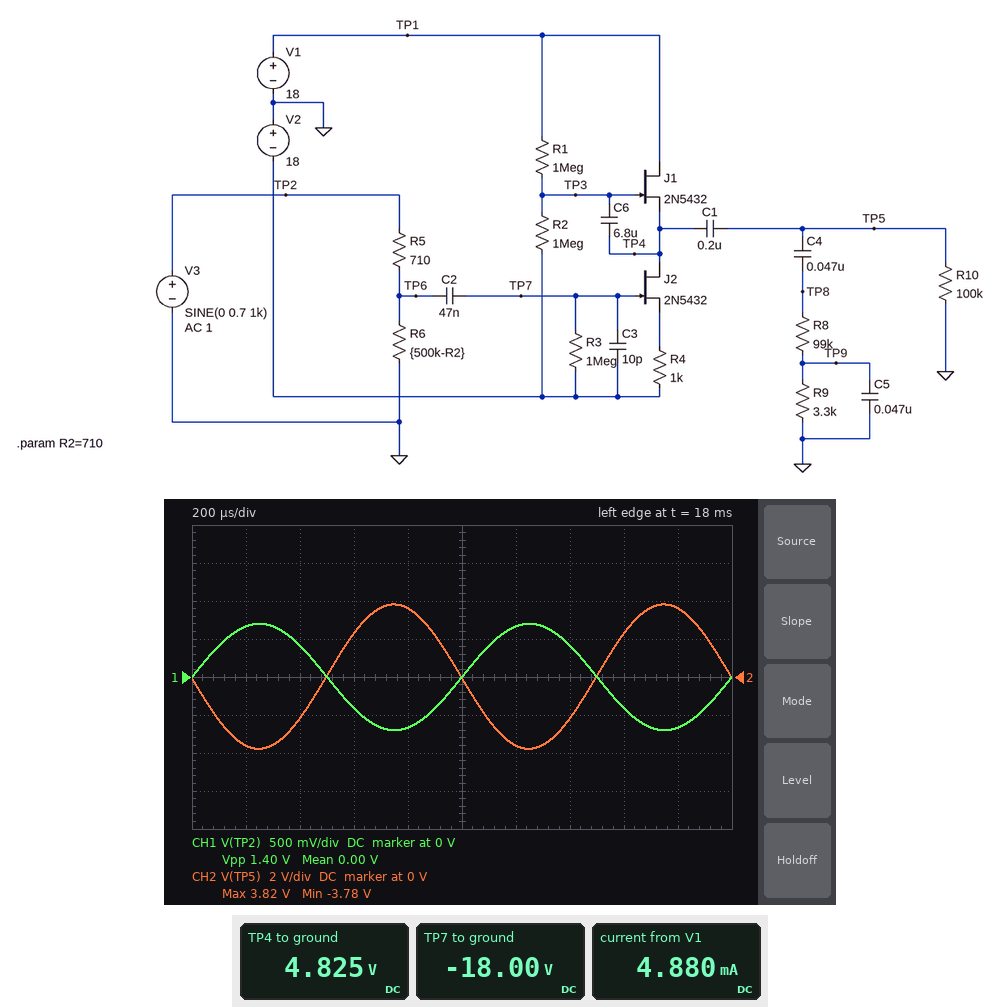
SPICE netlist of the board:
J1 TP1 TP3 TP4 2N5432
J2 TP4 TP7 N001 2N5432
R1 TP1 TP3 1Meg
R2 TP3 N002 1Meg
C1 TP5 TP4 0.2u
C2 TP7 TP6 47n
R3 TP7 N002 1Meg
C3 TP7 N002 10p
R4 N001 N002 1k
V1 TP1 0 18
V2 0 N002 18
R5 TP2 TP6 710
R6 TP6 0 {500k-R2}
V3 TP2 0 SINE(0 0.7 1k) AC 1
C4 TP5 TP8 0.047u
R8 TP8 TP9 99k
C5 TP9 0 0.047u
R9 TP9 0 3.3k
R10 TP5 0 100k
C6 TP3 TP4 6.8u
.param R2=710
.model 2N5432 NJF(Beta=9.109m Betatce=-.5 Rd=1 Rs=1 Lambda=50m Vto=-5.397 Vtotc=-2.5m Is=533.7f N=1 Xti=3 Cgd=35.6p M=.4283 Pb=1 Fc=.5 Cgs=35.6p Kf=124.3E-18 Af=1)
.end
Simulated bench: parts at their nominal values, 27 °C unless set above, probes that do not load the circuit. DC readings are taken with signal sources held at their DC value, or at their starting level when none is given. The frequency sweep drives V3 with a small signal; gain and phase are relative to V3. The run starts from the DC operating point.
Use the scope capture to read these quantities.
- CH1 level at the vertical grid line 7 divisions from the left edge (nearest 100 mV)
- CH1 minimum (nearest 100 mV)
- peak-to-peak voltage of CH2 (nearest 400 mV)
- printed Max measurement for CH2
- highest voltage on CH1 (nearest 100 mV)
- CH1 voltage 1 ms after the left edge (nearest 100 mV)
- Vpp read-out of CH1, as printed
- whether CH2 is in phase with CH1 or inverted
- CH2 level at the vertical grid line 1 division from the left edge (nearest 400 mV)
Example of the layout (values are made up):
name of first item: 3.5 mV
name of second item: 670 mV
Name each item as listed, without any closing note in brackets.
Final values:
CH1 level at the vertical grid line 7 divisions from the left edge: 400 mV
CH1 minimum: -700 mV
peak-to-peak voltage of CH2: 7.6 V
printed Max measurement for CH2: 3.82 V
highest voltage on CH1: 700 mV
CH1 voltage 1 ms after the left edge: 0 V
Vpp read-out of CH1, as printed: 1.40 V
whether CH2 is in phase with CH1 or inverted: inverted
CH2 level at the vertical grid line 1 division from the left edge: -3.6 V
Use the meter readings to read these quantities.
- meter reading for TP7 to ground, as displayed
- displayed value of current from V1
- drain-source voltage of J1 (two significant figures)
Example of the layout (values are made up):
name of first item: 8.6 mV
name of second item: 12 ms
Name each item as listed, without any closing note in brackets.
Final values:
meter reading for TP7 to ground, as displayed: -18.00 V
displayed value of current from V1: 4.880 mA
drain-source voltage of J1: 13 V
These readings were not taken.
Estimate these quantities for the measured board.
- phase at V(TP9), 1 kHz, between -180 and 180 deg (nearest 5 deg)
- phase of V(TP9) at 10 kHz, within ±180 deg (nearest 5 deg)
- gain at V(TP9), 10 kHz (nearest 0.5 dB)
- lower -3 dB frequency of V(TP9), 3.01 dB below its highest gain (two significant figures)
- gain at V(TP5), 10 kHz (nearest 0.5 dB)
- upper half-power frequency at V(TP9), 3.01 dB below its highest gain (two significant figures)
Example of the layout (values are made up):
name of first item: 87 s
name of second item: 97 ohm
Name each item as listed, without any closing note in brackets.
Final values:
phase at V(TP9), 1 kHz, between -180 and 180 deg: 140 deg
phase of V(TP9) at 10 kHz, within ±180 deg: 95 deg
gain at V(TP9), 10 kHz: -34.5 dB
lower -3 dB frequency of V(TP9), 3.01 dB below its highest gain: 38 Hz
gain at V(TP5), 10 kHz: 14.5 dB
upper half-power frequency at V(TP9), 3.01 dB below its highest gain: 1.1 kHz
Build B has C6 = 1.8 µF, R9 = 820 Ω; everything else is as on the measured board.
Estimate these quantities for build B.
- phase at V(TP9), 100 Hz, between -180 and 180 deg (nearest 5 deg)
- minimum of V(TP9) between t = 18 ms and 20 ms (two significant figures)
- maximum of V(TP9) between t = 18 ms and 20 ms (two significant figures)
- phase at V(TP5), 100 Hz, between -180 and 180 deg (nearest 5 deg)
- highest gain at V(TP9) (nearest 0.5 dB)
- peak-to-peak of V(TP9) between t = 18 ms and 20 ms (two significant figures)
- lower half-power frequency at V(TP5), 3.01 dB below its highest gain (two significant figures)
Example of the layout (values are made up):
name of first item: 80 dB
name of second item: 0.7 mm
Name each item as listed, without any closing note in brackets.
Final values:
phase at V(TP9), 100 Hz, between -180 and 180 deg: -145 deg
minimum of V(TP9) between t = 18 ms and 20 ms: -30 mV
maximum of V(TP9) between t = 18 ms and 20 ms: 30 mV
phase at V(TP5), 100 Hz, between -180 and 180 deg: -160 deg
highest gain at V(TP9): -27.0 dB
peak-to-peak of V(TP9) between t = 18 ms and 20 ms: 61 mV
lower half-power frequency at V(TP5), 3.01 dB below its highest gain: 25 Hz
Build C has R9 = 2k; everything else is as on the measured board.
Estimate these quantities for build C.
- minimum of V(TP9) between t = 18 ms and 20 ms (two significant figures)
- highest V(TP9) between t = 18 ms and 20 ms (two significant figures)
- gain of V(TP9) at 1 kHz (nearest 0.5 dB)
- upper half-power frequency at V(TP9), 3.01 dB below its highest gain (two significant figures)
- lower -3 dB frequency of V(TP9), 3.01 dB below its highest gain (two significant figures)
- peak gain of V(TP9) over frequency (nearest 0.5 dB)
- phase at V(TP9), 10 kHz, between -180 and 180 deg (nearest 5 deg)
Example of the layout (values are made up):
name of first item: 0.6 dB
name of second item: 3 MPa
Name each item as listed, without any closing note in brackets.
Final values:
minimum of V(TP9) between t = 18 ms and 20 ms: -65 mV
highest V(TP9) between t = 18 ms and 20 ms: 65 mV
gain of V(TP9) at 1 kHz: -20.5 dB
upper half-power frequency at V(TP9), 3.01 dB below its highest gain: 1.8 kHz
lower -3 dB frequency of V(TP9), 3.01 dB below its highest gain: 39 Hz
peak gain of V(TP9) over frequency: -19.5 dB
phase at V(TP9), 10 kHz, between -180 and 180 deg: 100 deg
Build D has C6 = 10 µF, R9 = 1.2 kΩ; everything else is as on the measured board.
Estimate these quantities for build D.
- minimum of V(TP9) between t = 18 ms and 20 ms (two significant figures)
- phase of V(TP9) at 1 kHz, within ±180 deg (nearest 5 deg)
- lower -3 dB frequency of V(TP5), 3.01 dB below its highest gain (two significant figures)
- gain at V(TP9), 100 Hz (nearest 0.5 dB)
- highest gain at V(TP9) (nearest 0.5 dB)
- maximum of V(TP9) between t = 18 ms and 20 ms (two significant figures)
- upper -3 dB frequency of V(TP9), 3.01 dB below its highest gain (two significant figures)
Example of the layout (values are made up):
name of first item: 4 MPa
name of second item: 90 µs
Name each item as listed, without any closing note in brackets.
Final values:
minimum of V(TP9) between t = 18 ms and 20 ms: -43 mV
phase of V(TP9) at 1 kHz, within ±180 deg: 165 deg
lower -3 dB frequency of V(TP5), 3.01 dB below its highest gain: 11 Hz
gain at V(TP9), 100 Hz: -24.5 dB
highest gain at V(TP9): -24.0 dB
maximum of V(TP9) between t = 18 ms and 20 ms: 43 mV
upper -3 dB frequency of V(TP9), 3.01 dB below its highest gain: 2.9 kHz
